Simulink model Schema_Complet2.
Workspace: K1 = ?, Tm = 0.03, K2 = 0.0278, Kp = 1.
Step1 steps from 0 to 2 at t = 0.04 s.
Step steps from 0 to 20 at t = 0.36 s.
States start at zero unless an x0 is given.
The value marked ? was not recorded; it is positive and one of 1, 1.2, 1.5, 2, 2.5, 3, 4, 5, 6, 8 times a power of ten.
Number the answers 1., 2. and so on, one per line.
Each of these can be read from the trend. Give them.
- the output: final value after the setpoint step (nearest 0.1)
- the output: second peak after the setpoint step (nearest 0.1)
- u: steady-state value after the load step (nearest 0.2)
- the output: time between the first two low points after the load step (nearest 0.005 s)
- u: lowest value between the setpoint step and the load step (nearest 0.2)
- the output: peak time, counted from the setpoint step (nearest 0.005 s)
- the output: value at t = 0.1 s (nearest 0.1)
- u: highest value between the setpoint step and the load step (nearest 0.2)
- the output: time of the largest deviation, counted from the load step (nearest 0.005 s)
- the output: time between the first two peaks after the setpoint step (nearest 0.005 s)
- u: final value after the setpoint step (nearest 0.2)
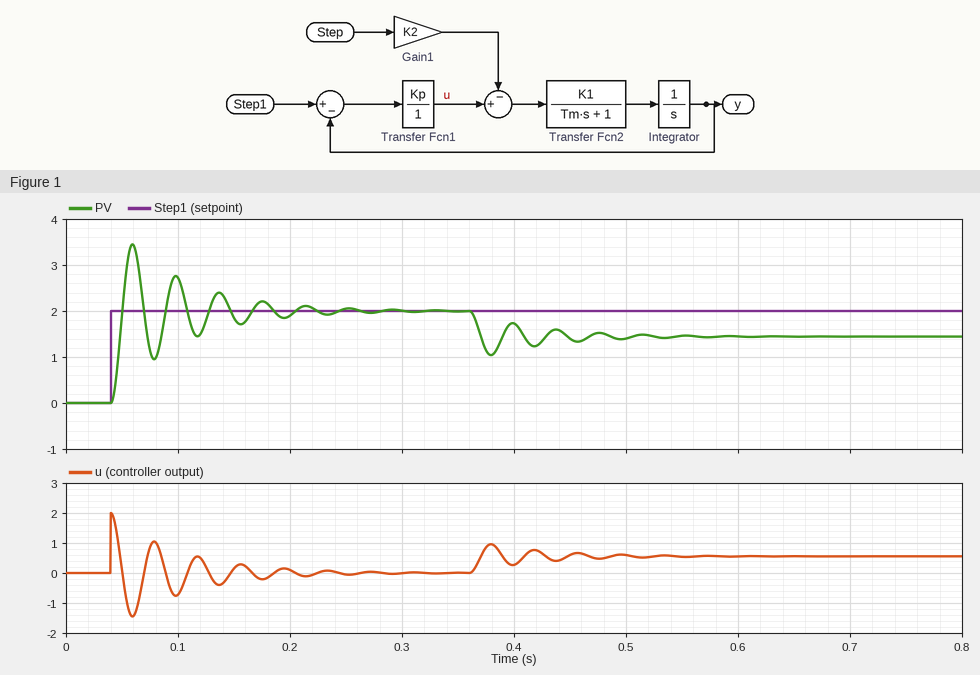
1. 2.0
2. 2.8
3. 0.6
4. 0.040 s
5. -1.4
6. 0.020 s
7. 2.7
8. 2.0
9. 0.020 s
10. 0.040 s
11. 0.0
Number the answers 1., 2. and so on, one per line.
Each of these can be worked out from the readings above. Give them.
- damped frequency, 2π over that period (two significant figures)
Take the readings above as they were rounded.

1. 160 rad/s
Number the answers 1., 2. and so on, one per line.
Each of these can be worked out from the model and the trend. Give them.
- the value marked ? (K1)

1. 800
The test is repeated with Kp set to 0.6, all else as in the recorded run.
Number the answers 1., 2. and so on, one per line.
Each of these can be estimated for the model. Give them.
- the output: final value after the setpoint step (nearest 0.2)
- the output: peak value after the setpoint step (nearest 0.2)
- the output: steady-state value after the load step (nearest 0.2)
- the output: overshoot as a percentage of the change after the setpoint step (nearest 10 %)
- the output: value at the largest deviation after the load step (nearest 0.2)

1. 2.0
2. 3.4
3. 1.0
4. 70 %
5. 0.4
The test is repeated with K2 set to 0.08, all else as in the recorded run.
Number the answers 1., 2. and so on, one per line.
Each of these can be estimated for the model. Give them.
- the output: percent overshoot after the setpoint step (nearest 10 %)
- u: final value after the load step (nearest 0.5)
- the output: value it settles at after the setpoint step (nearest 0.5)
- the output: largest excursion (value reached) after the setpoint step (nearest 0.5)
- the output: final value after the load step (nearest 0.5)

1. 70 %
2. 1.5
3. 2.0
4. 3.5
5. 0.5
